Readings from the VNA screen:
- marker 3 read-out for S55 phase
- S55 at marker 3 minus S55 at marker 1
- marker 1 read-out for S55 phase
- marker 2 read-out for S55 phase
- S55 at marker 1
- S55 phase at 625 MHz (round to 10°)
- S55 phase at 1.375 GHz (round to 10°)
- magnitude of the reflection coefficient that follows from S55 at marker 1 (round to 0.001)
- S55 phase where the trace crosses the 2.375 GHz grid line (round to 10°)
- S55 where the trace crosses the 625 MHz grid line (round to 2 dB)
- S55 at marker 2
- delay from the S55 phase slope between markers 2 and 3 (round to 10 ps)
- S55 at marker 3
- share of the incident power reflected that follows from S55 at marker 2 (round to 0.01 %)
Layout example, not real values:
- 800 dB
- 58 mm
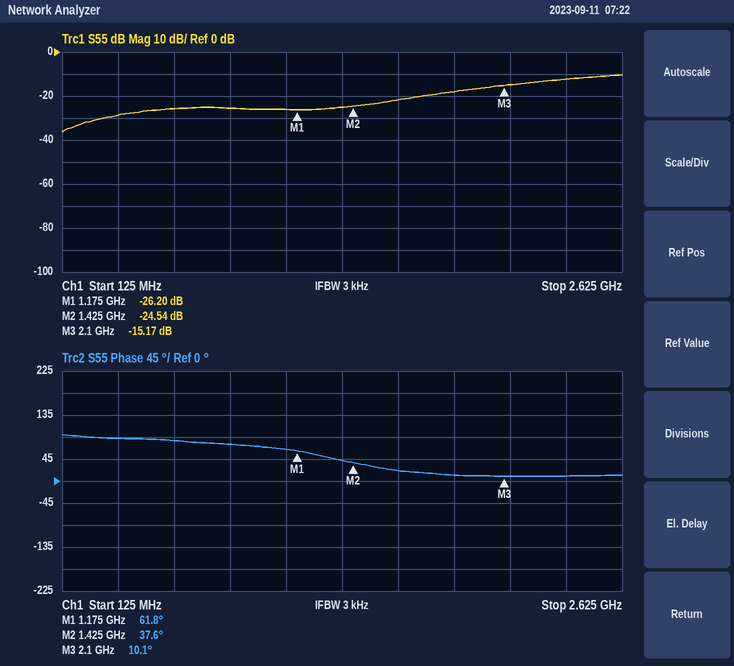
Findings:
- 10.1°
- 11.03 dB
- 61.8°
- 37.6°
- -26.20 dB
- 80°
- 40°
- 0.049
- 10°
- -26 dB
- -24.54 dB
- 110 ps
- -15.17 dB
- 0.35 %
